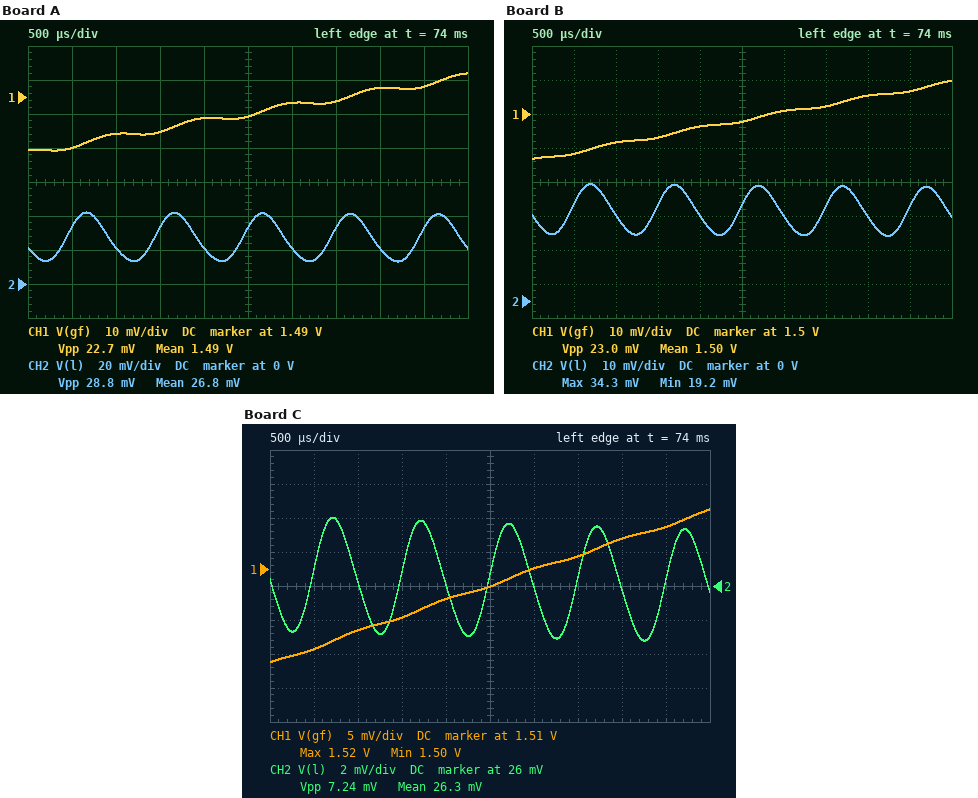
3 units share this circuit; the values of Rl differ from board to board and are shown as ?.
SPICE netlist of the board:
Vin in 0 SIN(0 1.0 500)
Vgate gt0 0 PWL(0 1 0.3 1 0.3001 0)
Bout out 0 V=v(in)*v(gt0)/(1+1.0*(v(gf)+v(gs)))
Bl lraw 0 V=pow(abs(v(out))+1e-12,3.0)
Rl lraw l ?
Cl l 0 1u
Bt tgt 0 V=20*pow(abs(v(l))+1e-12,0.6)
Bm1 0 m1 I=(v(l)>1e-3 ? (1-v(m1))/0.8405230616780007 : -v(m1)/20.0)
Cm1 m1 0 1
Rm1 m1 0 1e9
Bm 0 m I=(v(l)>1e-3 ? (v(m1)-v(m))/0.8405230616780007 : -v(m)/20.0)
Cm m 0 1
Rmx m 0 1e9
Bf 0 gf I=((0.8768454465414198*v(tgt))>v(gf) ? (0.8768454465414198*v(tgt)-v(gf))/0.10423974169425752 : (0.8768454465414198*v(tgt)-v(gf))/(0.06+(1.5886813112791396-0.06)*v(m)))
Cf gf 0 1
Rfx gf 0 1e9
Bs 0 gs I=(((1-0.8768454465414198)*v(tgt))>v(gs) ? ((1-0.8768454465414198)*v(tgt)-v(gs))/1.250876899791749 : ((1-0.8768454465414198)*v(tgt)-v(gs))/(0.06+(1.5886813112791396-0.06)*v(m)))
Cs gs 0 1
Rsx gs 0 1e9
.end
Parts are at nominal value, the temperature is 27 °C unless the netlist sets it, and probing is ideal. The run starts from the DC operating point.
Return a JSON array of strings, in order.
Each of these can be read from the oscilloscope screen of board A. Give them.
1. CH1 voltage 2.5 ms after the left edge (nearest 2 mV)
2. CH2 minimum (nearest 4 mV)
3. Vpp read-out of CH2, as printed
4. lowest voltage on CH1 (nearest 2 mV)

["1.484 V", "12 mV", "28.8 mV", "1.474 V"]
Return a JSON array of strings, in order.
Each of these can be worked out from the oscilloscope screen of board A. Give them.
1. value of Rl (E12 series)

["330 Ω"]
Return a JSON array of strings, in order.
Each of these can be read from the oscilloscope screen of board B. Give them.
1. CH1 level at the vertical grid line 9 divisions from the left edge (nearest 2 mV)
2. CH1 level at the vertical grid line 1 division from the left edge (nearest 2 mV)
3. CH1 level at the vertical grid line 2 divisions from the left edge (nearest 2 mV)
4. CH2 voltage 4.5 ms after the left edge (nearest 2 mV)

["1.506 V", "1.488 V", "1.492 V", "28 mV"]
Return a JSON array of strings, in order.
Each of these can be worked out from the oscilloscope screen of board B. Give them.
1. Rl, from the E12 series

["680 Ω"]
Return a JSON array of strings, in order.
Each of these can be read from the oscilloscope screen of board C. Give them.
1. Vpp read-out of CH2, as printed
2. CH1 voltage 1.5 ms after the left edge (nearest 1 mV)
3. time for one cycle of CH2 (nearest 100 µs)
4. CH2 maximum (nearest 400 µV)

["7.24 mV", "1.503 V", "1.0 ms", "30.0 mV"]
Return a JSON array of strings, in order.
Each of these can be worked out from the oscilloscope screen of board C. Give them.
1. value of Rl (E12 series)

["1.5 kΩ"]
